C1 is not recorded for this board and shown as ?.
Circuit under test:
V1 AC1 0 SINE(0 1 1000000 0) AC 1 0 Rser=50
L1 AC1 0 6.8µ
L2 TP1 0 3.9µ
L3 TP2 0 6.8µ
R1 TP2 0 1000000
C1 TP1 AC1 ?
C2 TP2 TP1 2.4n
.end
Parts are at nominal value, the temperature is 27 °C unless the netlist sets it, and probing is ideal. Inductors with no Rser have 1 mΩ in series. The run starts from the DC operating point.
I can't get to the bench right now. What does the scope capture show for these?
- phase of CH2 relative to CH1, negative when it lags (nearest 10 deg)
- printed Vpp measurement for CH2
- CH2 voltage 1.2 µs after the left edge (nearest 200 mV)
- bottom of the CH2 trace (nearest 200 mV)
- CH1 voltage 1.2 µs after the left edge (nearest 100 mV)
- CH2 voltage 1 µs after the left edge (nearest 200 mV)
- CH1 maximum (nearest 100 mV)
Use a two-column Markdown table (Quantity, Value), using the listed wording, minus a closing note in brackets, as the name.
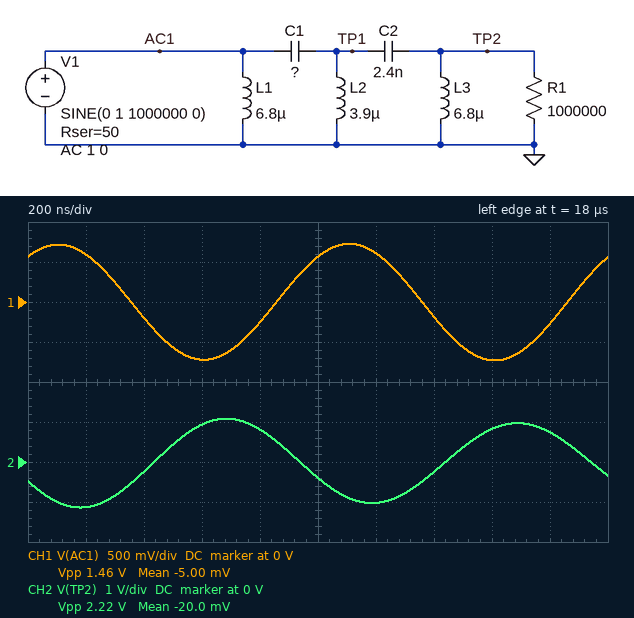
| Quantity | Value |
|---|---|
| phase of CH2 relative to CH1, negative when it lags | 150 deg |
| printed Vpp measurement for CH2 | 2.22 V |
| CH2 voltage 1.2 µs after the left edge | -1.0 V |
| bottom of the CH2 trace | -1.2 V |
| CH1 voltage 1.2 µs after the left edge | 600 mV |
| CH2 voltage 1 µs after the left edge | -400 mV |
| CH1 maximum | 700 mV |
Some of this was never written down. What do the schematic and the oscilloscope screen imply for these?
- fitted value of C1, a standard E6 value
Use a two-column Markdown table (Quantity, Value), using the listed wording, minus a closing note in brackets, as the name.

| Quantity | Value |
|---|---|
| fitted value of C1, a standard E6 value | 1 nF |
